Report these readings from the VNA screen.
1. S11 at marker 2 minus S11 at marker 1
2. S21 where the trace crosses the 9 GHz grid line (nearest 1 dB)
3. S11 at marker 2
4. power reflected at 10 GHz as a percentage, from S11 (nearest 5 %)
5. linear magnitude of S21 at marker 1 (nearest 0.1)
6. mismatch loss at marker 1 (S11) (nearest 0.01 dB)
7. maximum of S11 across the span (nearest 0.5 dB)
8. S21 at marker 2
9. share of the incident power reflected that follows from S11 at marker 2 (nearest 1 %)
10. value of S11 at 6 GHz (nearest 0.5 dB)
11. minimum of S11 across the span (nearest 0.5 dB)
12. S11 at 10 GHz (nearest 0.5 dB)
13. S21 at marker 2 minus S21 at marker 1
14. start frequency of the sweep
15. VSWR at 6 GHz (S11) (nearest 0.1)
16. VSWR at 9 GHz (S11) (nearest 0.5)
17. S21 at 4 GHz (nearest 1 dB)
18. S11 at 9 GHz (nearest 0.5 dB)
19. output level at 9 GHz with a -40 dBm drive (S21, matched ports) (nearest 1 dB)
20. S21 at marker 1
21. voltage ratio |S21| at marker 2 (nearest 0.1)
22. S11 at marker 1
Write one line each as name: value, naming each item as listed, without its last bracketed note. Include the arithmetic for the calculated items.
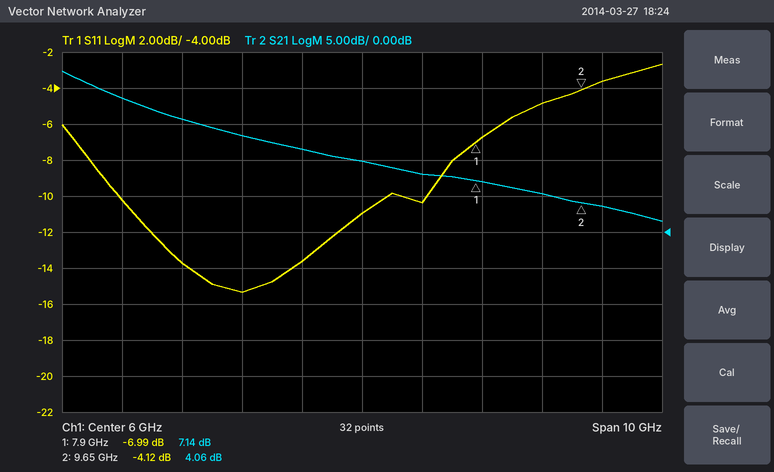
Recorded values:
S11 at marker 2 minus S11 at marker 1: -4.12 − (-6.99) = 2.87 dB
S21 where the trace crosses the 9 GHz grid line: 5 dB
S11 at marker 2: -4.12 dB
power reflected at 10 GHz as a percentage, from S11: 10^(-3.5/10) ≈ 45 %
linear magnitude of S21 at marker 1: 10^(7.14/20) ≈ 2.3
mismatch loss at marker 1 (S11): −10 log10(1 − 10^(-6.99/10)) ≈ 0.97 dB
maximum of S11 across the span: -2.5 dB
S21 at marker 2: 4.06 dB
share of the incident power reflected that follows from S11 at marker 2: 10^(-4.12/10) ≈ 39 %
value of S11 at 6 GHz: -11.0 dB
minimum of S11 across the span: -15.5 dB
S11 at 10 GHz: -3.5 dB
S21 at marker 2 minus S21 at marker 1: 4.06 − (7.14) = -3.08 dB
start frequency of the sweep: 1 GHz
VSWR at 6 GHz (S11): |Γ| = 10^(-11/20) = 0.2818; VSWR = (1 + 0.2818)/(1 − 0.2818) ≈ 1.8
VSWR at 9 GHz (S11): |Γ| = 10^(-5/20) = 0.5623; VSWR = (1 + 0.5623)/(1 − 0.5623) ≈ 3.57, so 3.5 to the nearest 0.5
S21 at 4 GHz: 13 dB
S11 at 9 GHz: -5.0 dB
output level at 9 GHz with a -40 dBm drive (S21, matched ports): -40 dBm + (5 dB) = -35 dBm
S21 at marker 1: 7.14 dB
voltage ratio |S21| at marker 2: 10^(4.06/20) ≈ 1.6
S11 at marker 1: -6.99 dB
